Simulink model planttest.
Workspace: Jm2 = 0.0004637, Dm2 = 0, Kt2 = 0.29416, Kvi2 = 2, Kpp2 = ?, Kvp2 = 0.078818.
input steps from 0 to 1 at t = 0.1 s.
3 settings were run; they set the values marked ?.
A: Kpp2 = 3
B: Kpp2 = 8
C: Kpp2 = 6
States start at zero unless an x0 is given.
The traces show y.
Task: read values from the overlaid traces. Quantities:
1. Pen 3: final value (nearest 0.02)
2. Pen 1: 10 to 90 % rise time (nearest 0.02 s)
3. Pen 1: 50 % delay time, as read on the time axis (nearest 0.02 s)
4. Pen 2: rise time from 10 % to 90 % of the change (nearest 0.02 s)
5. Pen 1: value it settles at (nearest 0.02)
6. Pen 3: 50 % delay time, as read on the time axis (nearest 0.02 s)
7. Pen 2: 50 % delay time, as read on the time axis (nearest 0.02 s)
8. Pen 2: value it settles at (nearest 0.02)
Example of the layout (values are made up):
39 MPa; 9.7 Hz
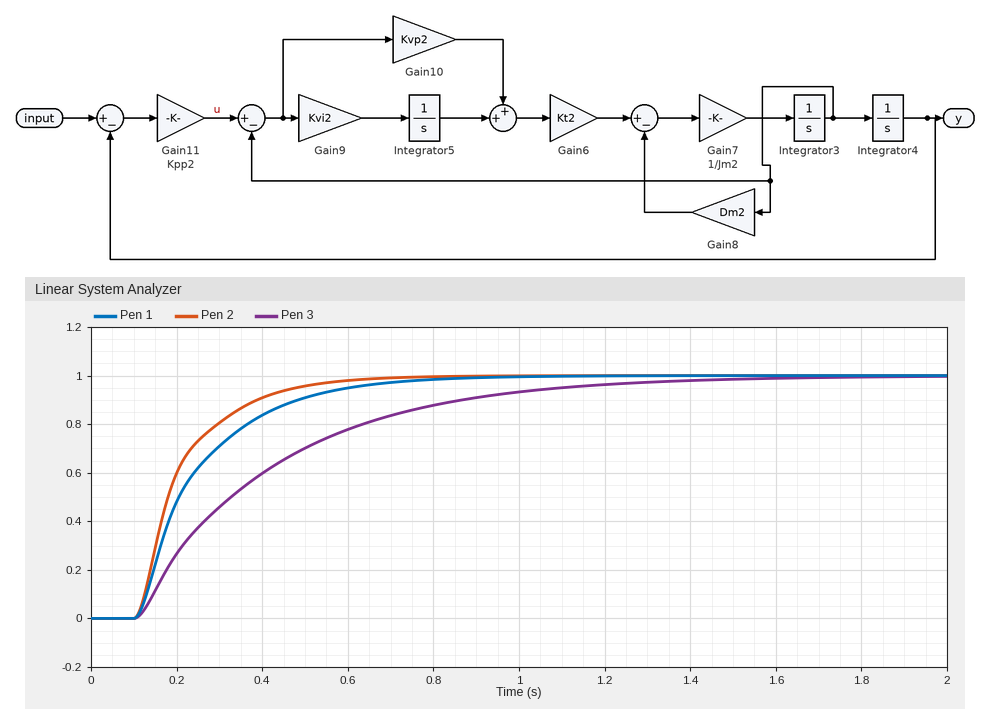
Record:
1.00; 0.36 s; 0.20 s; 0.26 s; 1.00; 0.32 s; 0.18 s; 1.00
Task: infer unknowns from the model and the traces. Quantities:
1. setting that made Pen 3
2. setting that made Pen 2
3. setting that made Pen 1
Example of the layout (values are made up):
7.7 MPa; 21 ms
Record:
A; B; C
